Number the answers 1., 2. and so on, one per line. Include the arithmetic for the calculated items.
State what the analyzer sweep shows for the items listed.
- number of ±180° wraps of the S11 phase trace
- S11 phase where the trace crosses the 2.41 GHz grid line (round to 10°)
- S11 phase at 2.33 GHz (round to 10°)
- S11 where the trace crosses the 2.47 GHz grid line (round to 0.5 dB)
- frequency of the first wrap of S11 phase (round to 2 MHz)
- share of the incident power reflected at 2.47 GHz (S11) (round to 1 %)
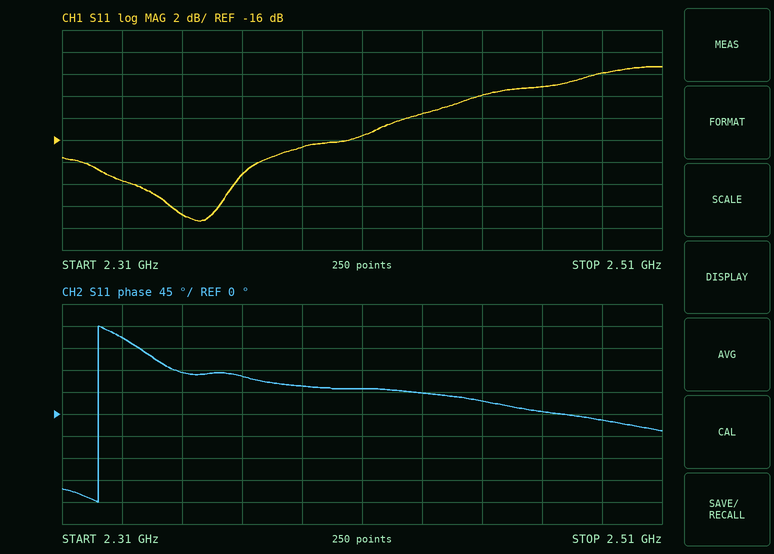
1. 1
2. 50°
3. 160°
4. -11.0 dB
5. 2.322 GHz
6. 10^(-11/10) ≈ 8 %
